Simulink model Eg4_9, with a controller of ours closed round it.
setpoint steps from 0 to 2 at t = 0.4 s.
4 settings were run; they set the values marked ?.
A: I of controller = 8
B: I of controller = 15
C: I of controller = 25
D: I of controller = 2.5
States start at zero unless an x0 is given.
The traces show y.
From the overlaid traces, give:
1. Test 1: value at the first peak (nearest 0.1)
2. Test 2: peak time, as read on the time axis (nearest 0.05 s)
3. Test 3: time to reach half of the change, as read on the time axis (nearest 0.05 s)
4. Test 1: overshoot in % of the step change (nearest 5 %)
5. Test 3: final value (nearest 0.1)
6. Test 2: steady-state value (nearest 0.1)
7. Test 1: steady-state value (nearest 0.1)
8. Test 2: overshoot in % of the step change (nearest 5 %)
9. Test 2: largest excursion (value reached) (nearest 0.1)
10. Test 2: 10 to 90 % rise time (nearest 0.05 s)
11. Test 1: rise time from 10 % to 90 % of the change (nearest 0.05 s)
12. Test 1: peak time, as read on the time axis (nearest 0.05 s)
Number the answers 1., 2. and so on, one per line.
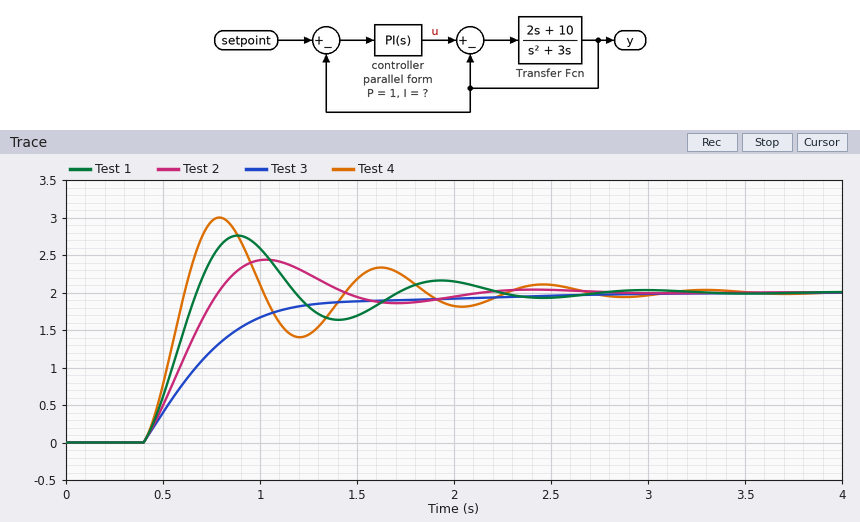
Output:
1. 2.8
2. 1.05 s
3. 0.65 s
4. 40 %
5. 2.0
6. 2.0
7. 2.0
8. 20 %
9. 2.4
10. 0.30 s
11. 0.20 s
12. 0.90 s
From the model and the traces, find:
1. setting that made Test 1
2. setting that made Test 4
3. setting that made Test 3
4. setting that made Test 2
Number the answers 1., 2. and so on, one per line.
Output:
1. B
2. C
3. D
4. A
